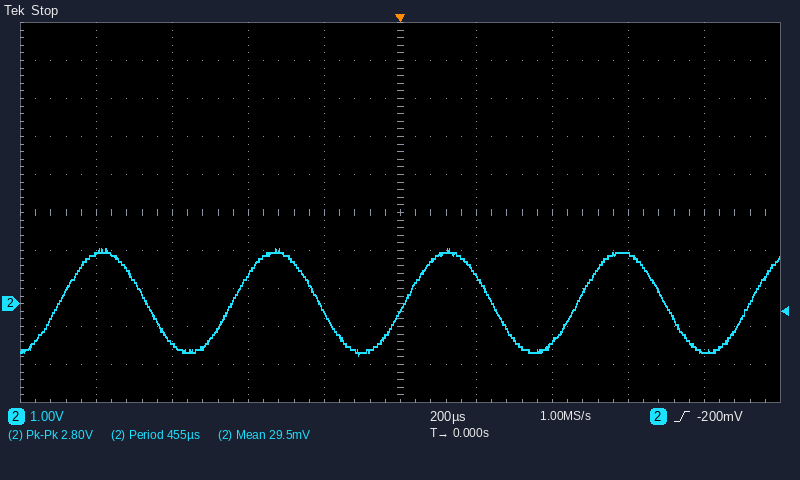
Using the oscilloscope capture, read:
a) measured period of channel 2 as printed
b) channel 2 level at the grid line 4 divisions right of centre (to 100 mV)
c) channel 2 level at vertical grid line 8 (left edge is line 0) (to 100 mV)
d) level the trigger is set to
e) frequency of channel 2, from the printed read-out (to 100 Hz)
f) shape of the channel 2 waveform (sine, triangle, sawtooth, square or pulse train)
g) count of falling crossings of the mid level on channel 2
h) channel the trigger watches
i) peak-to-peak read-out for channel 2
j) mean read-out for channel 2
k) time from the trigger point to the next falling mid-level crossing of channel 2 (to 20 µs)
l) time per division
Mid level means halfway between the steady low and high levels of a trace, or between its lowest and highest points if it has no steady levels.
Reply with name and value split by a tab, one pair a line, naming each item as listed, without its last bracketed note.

measured period of channel 2 as printed	455 µs
channel 2 level at the grid line 4 divisions right of centre	-1.2 V
channel 2 level at vertical grid line 8 (left edge is line 0)	1.3 V
level the trigger is set to	-200 mV
frequency of channel 2, from the printed read-out	2.2 kHz
shape of the channel 2 waveform	sine
count of falling crossings of the mid level on channel 2	4
channel the trigger watches	channel 2
peak-to-peak read-out for channel 2	2.80 V
mean read-out for channel 2	29.5 mV
time from the trigger point to the next falling mid-level crossing of channel 2	240 µs
time per division	200 µs
